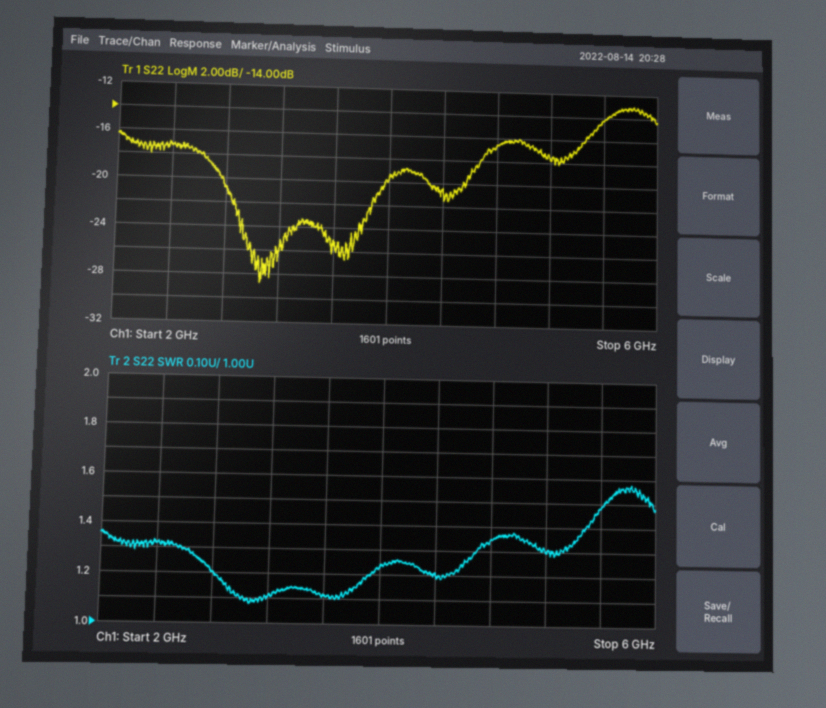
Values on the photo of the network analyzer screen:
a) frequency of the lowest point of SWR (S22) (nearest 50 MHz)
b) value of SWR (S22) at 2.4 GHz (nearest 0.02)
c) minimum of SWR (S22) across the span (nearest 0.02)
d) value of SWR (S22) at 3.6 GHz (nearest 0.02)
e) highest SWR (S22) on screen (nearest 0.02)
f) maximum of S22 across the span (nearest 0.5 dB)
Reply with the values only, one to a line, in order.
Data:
3.05 GHz
1.32
1.08
1.12
1.58
-13.0 dB
